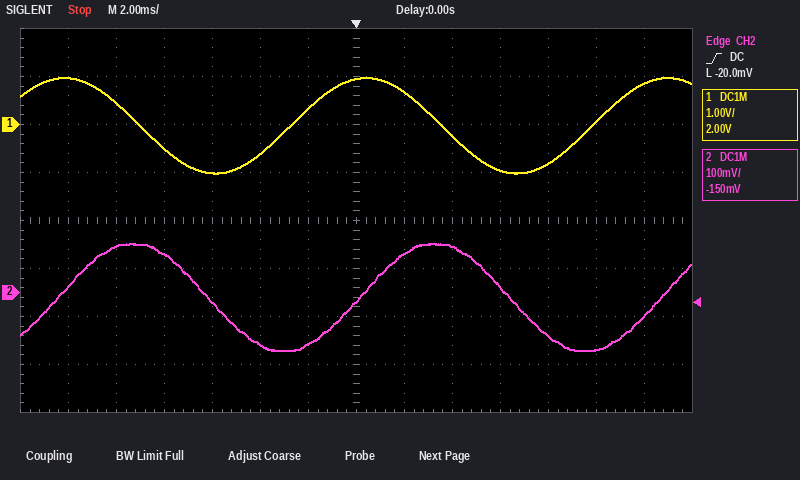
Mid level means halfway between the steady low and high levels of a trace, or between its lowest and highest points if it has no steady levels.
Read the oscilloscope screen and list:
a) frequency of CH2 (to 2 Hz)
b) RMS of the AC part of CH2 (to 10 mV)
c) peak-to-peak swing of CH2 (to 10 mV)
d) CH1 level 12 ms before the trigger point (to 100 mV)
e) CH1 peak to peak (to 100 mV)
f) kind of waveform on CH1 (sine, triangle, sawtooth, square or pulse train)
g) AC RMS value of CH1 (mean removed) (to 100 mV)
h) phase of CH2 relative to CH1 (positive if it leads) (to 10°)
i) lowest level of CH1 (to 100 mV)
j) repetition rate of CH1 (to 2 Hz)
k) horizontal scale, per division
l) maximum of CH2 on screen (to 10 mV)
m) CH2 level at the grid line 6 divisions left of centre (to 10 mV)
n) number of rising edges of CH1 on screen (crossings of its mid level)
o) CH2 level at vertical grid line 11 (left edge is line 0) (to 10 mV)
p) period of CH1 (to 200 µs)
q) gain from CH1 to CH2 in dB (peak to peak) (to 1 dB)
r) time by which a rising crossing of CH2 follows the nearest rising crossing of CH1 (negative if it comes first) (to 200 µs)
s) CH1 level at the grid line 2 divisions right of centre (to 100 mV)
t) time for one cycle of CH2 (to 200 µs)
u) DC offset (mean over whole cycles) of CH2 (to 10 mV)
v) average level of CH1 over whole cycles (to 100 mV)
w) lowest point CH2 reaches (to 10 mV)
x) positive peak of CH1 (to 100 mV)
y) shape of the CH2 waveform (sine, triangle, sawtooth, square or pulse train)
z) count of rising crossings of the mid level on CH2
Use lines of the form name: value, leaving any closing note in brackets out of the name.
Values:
frequency of CH2: 80 Hz
RMS of the AC part of CH2: 80 mV
peak-to-peak swing of CH2: 220 mV
CH1 level 12 ms before the trigger point: 1.0 V
CH1 peak to peak: 2.0 V
kind of waveform on CH1: sine
AC RMS value of CH1 (mean removed): 700 mV
phase of CH2 relative to CH1 (positive if it leads): -80°
lowest level of CH1: -1.0 V
repetition rate of CH1: 80 Hz
horizontal scale, per division: 2 ms
maximum of CH2 on screen: 100 mV
CH2 level at the grid line 6 divisions left of centre: 10 mV
number of rising edges of CH1 on screen: 2
CH2 level at vertical grid line 11 (left edge is line 0): -90 mV
period of CH1: 12.6 ms
gain from CH1 to CH2 in dB (peak to peak): -19 dB
time by which a rising crossing of CH2 follows the nearest rising crossing of CH1 (negative if it comes first): +2.8 ms
CH1 level at the grid line 2 divisions right of centre: -200 mV
time for one cycle of CH2: 12.6 ms
DC offset (mean over whole cycles) of CH2: -10 mV
average level of CH1 over whole cycles: 0.0 V
lowest point CH2 reaches: -120 mV
positive peak of CH1: 1.0 V
shape of the CH2 waveform: sine
count of rising crossings of the mid level on CH2: 3
